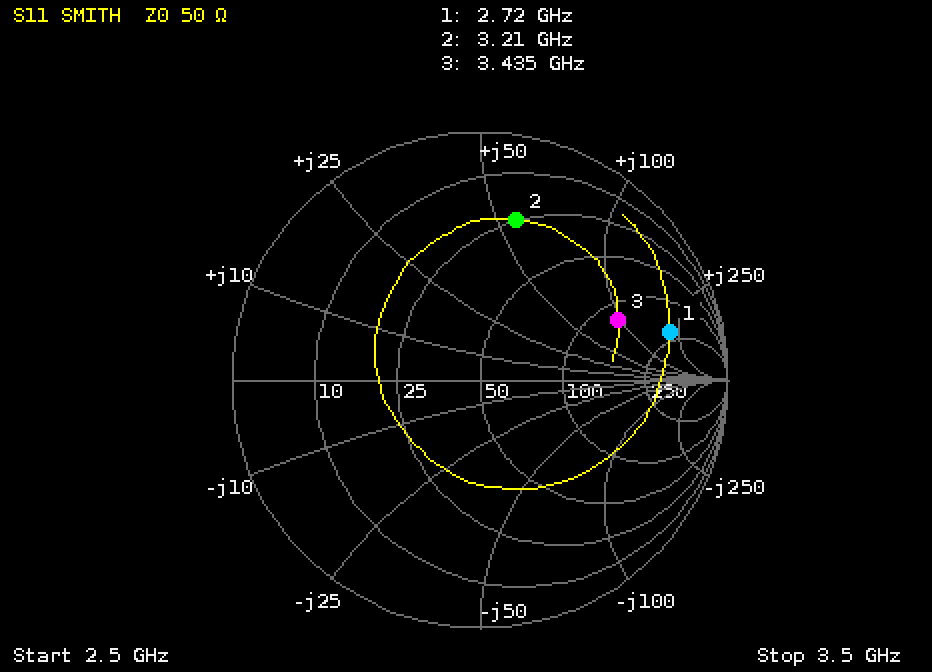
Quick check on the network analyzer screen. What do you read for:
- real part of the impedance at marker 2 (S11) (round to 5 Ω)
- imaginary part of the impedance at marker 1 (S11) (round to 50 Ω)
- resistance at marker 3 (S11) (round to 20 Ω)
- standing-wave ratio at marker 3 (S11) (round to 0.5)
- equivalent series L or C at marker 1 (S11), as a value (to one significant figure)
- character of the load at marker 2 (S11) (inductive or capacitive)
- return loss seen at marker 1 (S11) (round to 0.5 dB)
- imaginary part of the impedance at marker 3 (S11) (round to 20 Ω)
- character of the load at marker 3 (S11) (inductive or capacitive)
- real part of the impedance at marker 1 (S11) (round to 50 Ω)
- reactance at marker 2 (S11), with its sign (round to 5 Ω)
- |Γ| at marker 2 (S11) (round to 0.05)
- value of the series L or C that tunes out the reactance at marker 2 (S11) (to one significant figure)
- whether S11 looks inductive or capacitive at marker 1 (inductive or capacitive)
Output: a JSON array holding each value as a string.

["25 Ω", "+200 Ω", "120 Ω", "4.0", "10 nH", "inductive", "2.0 dB", "+100 Ω", "inductive", "200 Ω", "+55 Ω", "0.65", "900 fF", "inductive"]
